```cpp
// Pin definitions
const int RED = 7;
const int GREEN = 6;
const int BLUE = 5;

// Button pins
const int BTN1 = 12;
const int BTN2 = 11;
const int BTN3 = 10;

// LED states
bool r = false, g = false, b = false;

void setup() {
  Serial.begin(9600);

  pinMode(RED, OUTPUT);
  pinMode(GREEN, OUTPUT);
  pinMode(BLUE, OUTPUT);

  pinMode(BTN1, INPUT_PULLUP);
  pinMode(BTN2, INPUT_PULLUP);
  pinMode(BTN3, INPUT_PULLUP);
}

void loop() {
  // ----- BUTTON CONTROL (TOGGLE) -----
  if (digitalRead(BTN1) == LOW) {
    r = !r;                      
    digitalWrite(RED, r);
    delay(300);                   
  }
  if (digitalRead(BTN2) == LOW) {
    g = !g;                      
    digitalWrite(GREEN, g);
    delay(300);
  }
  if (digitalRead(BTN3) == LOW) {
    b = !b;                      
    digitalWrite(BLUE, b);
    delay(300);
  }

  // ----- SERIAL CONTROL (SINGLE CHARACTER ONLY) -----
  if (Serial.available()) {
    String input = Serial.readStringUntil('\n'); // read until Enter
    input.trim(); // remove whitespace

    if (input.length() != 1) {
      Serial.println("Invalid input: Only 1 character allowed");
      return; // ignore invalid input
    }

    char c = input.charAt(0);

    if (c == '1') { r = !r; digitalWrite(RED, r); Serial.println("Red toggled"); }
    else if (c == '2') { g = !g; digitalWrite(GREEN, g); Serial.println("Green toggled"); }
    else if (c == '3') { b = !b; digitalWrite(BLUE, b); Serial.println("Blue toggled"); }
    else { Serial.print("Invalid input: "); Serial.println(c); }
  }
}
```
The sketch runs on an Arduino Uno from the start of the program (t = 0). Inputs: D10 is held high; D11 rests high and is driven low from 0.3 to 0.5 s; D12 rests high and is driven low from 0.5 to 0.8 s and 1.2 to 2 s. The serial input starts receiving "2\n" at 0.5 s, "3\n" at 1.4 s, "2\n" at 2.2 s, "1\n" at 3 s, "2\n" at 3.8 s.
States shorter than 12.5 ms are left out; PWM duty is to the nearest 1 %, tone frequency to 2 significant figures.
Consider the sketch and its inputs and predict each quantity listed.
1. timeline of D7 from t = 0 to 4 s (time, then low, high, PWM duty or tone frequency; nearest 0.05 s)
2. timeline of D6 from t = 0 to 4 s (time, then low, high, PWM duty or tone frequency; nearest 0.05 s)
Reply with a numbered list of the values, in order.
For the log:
1. 0 s low; 0.6 s high; 1.2 s low; 1.5 s high; 1.8 s low; 3 s high
2. 0 s low; 0.3 s high; 0.6 s low; 2.2 s high; 3.8 s low
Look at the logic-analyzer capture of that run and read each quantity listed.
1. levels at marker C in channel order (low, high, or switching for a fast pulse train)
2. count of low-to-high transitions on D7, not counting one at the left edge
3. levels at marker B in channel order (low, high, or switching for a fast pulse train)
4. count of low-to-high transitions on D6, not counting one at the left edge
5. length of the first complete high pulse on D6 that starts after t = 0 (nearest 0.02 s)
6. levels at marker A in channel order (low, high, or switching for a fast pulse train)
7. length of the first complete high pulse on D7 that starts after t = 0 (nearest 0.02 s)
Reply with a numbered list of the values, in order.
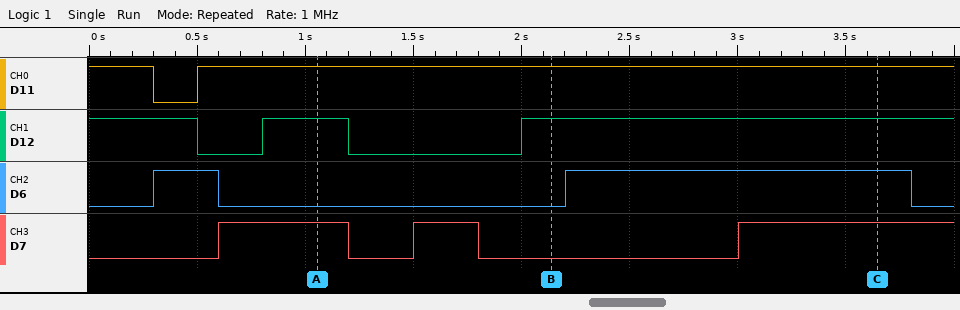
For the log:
1. D11 high, D12 high, D6 high, D7 high
2. 3
3. D11 high, D12 high, D6 low, D7 low
4. 2
5. 0.30 s
6. D11 high, D12 high, D6 low, D7 high
7. 0.60 s
